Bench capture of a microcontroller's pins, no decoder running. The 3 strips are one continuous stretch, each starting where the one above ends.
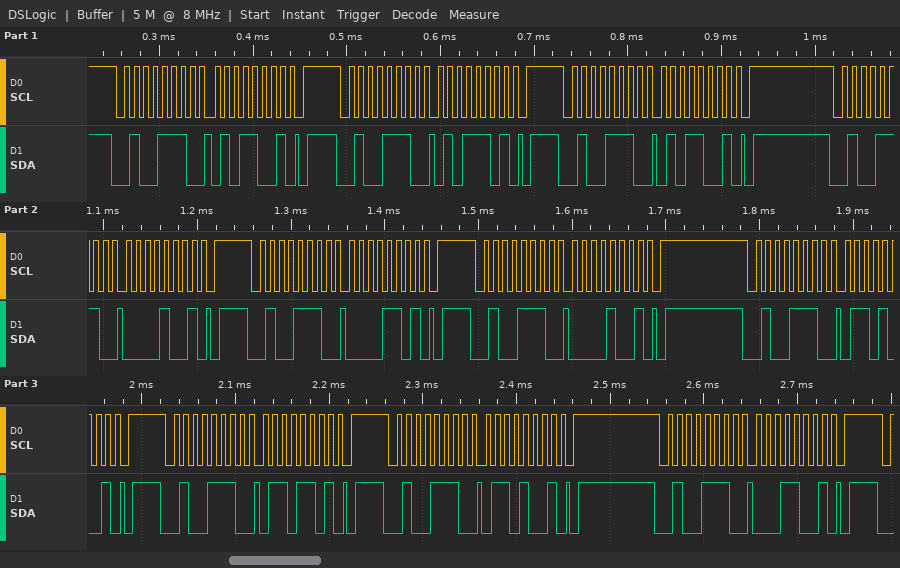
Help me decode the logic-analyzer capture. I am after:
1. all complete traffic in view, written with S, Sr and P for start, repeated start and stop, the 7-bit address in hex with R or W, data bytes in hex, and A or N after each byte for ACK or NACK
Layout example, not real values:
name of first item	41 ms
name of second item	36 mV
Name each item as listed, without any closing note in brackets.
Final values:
all complete traffic in view, written with S, Sr and P for start, repeated start and stop, the 7-bit address in hex with R or W, data bytes in hex, and A or N after each byte for ACK or NACK	S 27W A 59 A P S 27W A 5D A P S 27W A 59 A P S 27W A 09 A P S 27W A 0D A P S 27W A 09 A P S 27W A 69 A P S 27W A 6D A P S 27W A 69 A P S 27W A 19 A P
